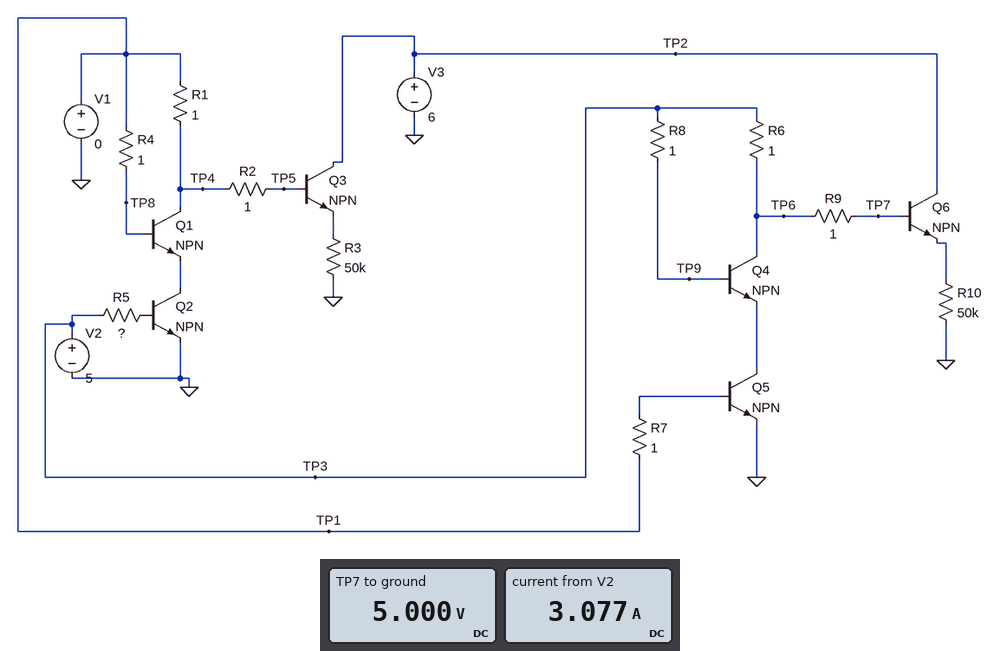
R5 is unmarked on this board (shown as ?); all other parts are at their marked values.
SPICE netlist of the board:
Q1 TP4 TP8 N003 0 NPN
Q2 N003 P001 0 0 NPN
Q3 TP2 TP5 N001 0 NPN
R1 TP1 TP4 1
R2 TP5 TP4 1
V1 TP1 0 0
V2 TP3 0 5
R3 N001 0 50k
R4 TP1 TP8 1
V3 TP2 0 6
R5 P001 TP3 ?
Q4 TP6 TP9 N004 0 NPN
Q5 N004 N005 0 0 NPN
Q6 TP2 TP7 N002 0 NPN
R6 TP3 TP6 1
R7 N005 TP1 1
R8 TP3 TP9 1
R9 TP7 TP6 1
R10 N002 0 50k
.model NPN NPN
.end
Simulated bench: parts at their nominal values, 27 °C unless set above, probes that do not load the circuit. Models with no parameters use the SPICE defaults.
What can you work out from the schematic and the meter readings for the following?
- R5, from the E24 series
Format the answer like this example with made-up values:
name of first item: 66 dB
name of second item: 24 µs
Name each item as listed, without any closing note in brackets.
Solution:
R5, from the E24 series: 1.3 Ω
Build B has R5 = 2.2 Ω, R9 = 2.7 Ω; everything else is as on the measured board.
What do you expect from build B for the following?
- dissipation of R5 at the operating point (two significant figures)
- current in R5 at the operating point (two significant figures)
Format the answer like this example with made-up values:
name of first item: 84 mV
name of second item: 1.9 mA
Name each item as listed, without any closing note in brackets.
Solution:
dissipation of R5 at the operating point: 7.3 W
current in R5 at the operating point: 1.8 A
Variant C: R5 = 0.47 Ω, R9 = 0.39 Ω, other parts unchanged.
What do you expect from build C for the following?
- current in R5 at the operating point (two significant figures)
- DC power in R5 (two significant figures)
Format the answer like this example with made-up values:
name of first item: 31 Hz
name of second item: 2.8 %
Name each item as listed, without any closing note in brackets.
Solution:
current in R5 at the operating point: 8.5 A
DC power in R5: 34 W
